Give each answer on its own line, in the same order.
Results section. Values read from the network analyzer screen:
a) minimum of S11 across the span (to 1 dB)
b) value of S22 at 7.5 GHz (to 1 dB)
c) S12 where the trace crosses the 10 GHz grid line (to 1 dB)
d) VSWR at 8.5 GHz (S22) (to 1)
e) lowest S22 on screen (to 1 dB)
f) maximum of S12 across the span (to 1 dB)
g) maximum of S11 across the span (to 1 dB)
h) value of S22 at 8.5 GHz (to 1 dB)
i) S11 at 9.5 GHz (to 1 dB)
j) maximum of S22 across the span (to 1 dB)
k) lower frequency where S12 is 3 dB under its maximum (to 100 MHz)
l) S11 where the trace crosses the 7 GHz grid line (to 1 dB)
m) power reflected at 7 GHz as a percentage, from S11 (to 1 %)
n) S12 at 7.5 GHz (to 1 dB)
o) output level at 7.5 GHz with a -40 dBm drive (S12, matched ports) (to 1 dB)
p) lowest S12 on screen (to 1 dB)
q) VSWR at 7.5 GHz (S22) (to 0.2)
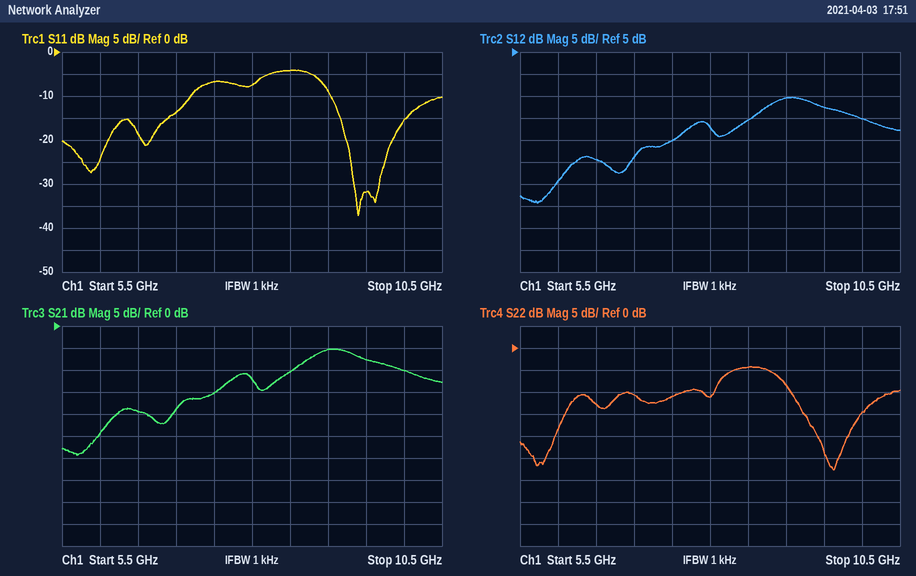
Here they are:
-37 dB
-11 dB
-10 dB
4
-28 dB
-5 dB
-4 dB
-4 dB
-32 dB
-4 dB
8.7 GHz
-14 dB
4 %
-15 dB
-55 dBm
-29 dB
1.8
